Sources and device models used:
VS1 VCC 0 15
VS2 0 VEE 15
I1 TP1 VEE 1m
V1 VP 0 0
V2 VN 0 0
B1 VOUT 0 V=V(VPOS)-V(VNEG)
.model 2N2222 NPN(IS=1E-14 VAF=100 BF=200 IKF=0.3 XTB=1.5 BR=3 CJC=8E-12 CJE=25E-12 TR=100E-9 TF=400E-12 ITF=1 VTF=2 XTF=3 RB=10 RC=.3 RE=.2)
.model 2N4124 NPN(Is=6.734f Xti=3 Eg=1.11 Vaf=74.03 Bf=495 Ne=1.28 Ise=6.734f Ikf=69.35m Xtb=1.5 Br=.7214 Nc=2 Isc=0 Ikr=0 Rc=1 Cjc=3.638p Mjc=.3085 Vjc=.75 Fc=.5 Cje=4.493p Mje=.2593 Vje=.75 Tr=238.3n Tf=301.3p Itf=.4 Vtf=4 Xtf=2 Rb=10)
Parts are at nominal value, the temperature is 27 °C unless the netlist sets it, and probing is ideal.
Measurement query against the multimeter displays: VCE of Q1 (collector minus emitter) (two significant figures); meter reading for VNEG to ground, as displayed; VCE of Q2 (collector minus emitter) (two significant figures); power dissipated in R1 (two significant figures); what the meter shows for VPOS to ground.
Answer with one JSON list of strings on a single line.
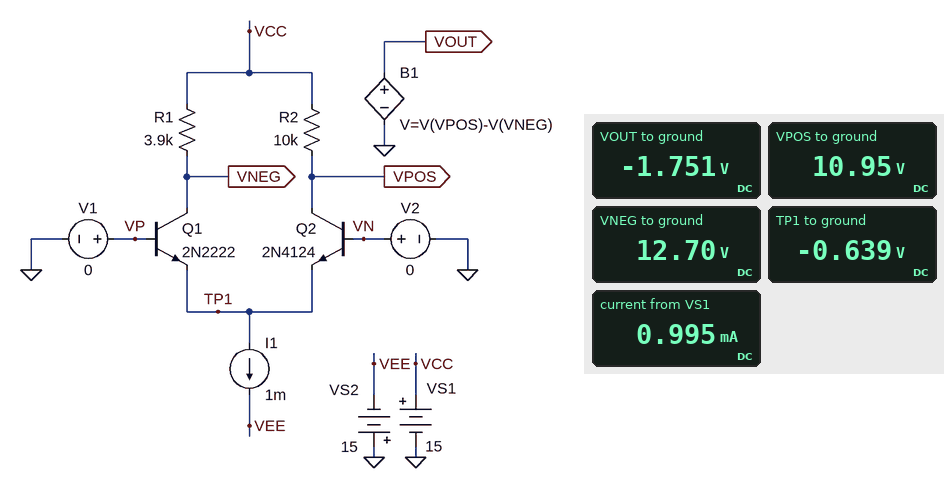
["13 V", "12.70 V", "12 V", "1.4 mW", "10.95 V"]
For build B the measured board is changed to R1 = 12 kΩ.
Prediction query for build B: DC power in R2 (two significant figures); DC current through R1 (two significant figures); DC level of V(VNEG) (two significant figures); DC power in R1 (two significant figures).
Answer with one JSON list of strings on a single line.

["1.7 mW", "580 µA", "8.0 V", "4.0 mW"]
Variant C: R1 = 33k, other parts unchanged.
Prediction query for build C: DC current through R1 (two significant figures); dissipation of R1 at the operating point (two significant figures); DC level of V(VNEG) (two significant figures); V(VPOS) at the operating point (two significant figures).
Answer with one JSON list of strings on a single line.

["470 µA", "7.4 mW", "-600 mV", "10 V"]
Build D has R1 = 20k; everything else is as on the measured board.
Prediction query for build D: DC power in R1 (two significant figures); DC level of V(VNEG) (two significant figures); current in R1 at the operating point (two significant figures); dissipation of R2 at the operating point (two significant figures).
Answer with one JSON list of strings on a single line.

["6.5 mW", "3.6 V", "570 µA", "1.8 mW"]
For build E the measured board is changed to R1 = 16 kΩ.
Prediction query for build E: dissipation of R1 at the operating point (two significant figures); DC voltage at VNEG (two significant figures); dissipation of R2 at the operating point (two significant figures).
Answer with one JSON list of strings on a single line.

["5.3 mW", "5.8 V", "1.8 mW"]
